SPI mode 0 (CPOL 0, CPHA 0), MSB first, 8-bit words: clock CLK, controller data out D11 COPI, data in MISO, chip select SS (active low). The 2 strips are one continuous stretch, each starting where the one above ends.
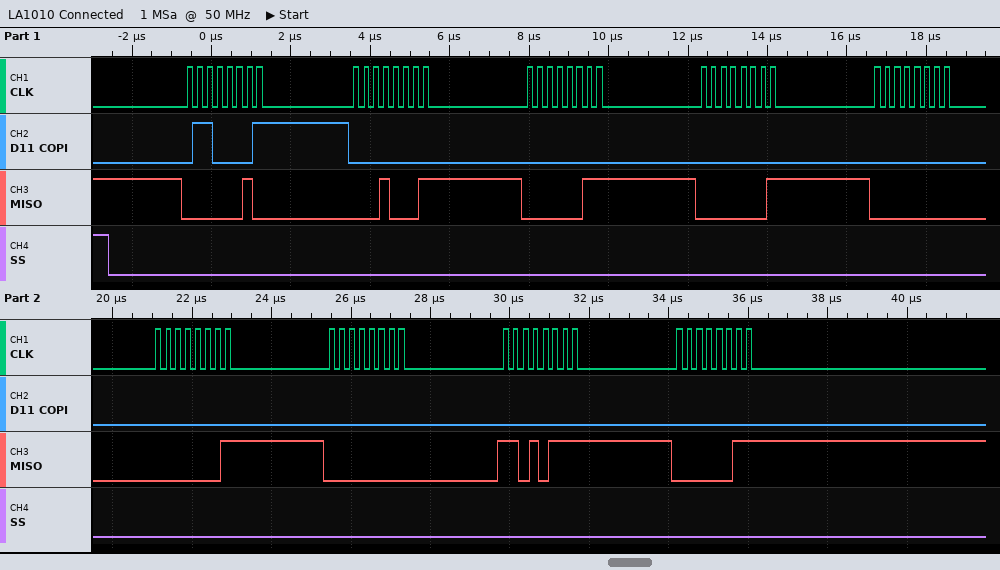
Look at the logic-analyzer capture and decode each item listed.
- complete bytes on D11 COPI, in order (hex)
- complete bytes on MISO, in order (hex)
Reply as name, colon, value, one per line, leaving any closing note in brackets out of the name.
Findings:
complete bytes on D11 COPI, in order: 61 00 00 00 00 00 00 00 00
complete bytes on MISO, in order: 02 11 03 01 00 01 00 D7 03
